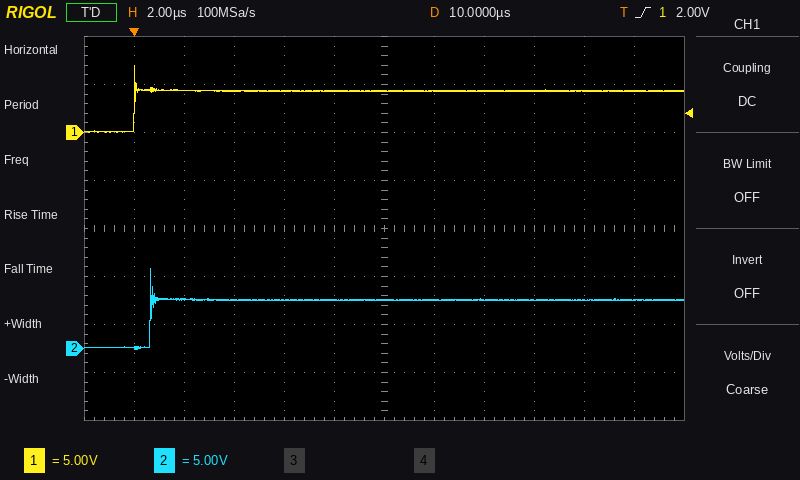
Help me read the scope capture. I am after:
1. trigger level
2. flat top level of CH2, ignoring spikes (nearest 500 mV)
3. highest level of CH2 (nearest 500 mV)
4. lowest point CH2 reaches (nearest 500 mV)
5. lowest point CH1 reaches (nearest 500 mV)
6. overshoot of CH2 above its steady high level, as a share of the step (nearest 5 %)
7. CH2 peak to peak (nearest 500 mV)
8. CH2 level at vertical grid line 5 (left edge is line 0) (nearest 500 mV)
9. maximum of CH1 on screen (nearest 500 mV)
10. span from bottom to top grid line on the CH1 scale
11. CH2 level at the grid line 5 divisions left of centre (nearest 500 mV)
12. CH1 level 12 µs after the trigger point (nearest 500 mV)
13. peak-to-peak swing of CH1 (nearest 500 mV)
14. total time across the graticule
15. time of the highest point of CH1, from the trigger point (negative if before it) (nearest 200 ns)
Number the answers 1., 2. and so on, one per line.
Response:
1. 2.00 V
2. 5.0 V
3. 8.5 V
4. 0.0 V
5. 0.0 V
6. 65 %
7. 8.5 V
8. 5.0 V
9. 7.0 V
10. 40 V
11. 0.0 V
12. 4.5 V
13. 7.0 V
14. 24 µs
15. 0.0 µs
